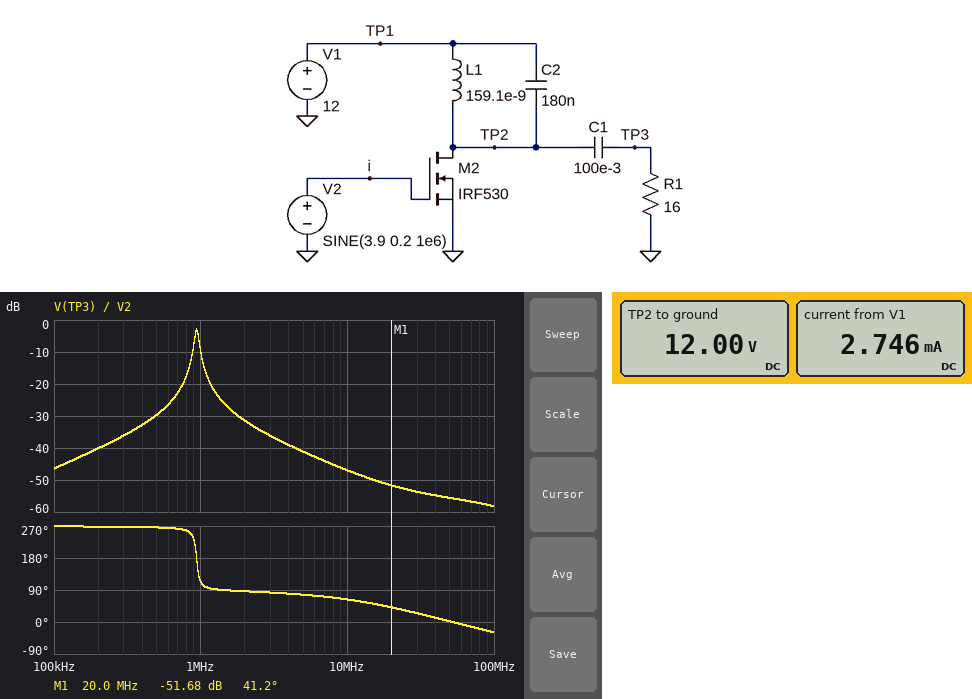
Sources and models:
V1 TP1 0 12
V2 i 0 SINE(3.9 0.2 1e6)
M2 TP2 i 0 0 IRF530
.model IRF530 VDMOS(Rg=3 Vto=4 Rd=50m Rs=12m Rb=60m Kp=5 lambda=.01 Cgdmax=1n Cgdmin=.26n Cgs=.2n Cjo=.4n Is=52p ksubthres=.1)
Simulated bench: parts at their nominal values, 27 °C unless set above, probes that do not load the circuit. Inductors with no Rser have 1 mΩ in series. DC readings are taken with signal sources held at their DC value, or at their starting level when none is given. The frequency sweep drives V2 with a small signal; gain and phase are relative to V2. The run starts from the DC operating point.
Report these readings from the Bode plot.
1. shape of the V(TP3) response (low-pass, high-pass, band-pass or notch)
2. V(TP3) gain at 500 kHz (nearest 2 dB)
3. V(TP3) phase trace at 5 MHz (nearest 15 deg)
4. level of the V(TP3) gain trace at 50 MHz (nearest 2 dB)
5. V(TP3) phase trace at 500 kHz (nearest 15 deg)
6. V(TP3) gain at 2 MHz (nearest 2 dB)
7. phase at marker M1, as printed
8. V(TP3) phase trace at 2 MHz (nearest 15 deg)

band-pass
-30 dB
75 deg
-56 dB
270 deg
-32 dB
41.2 deg
90 deg
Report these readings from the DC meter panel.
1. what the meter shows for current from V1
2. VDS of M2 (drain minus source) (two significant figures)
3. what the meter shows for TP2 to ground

2.746 mA
12 V
12.00 V
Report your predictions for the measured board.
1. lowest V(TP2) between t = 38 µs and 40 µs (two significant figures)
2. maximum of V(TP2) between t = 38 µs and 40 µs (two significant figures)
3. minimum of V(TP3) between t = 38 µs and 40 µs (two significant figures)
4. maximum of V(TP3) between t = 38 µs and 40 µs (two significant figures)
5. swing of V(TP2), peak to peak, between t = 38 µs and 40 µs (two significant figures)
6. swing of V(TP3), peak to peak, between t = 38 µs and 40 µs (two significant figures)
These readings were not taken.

12 V
12 V
-140 mV
130 mV
270 mV
270 mV
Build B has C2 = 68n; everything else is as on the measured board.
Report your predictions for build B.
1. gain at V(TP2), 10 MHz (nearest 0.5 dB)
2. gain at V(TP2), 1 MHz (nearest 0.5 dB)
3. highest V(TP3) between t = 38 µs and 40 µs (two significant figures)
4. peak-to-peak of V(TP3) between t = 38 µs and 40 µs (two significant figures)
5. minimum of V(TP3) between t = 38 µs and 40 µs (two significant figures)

-38.5 dB
-21.5 dB
59 mV
110 mV
-50 mV
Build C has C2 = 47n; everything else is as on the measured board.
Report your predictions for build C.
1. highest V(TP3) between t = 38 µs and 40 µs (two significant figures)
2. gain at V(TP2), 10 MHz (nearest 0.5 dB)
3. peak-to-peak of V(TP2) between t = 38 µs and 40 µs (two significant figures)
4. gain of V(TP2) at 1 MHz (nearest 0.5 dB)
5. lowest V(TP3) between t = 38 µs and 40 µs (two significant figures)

120 mV
-35.0 dB
220 mV
-23.5 dB
-98 mV
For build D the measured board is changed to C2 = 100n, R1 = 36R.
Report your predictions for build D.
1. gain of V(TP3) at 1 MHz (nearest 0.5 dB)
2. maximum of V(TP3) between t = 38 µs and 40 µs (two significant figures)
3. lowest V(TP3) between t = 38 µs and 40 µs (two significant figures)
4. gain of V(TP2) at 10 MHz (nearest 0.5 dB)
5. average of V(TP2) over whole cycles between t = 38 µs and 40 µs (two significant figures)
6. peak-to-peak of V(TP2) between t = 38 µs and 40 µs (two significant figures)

-18.0 dB
63 mV
-59 mV
-42.0 dB
12 V
120 mV
